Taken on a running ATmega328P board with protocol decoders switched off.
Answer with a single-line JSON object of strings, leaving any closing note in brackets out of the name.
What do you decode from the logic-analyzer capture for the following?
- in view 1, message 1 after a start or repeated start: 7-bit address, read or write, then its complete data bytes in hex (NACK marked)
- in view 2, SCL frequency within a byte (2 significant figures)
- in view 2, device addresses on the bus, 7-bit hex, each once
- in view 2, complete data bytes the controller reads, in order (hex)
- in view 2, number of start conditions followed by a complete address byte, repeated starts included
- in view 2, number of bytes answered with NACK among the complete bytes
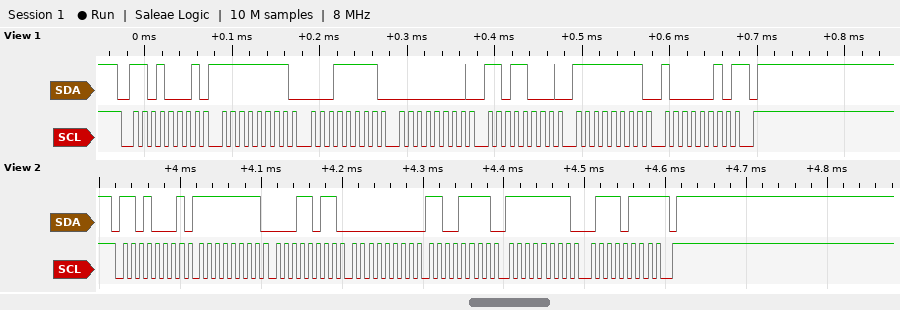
{"in view 1, message 1 after a start or repeated start: 7-bit address, read or write, then its complete data bytes in hex": "0x68 read: FF 1F 00 D8 FF 82 NACK", "in view 2, SCL frequency within a byte": "100 kHz", "in view 2, device addresses on the bus, 7-bit hex, each once": "0x68", "in view 2, complete data bytes the controller reads, in order": "FF 1B 00 CF FF 77", "in view 2, number of start conditions followed by a complete address byte, repeated starts included": "1", "in view 2, number of bytes answered with NACK among the complete bytes": "1"}
